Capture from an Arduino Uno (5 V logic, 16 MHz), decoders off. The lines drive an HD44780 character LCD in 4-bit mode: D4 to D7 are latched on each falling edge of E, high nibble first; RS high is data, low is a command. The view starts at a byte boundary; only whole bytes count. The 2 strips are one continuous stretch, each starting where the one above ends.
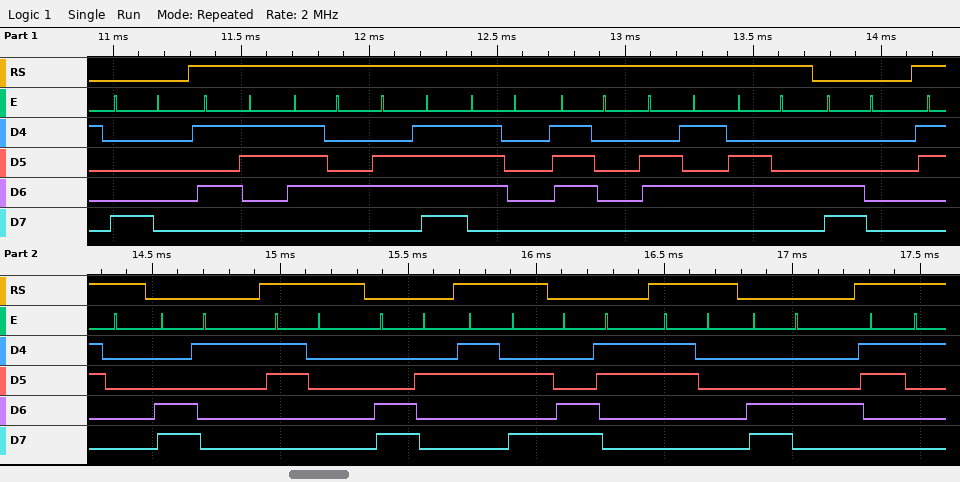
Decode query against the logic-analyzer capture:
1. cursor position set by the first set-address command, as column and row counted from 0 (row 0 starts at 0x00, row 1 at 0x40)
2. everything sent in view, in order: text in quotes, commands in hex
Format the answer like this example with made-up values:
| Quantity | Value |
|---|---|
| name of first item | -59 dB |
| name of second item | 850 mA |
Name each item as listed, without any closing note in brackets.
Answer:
| Quantity | Value |
|---|---|
| cursor position set by the first set-address command, as column and row counted from 0 | column 0, row 0 |
| everything sent in view, in order: text in quotes, commands in hex | 0x80 "Stopped" 0xC0 "0" 0xC1 "0" 0xC2 ":" 0xC3 "0" 0xC4 "1" |
